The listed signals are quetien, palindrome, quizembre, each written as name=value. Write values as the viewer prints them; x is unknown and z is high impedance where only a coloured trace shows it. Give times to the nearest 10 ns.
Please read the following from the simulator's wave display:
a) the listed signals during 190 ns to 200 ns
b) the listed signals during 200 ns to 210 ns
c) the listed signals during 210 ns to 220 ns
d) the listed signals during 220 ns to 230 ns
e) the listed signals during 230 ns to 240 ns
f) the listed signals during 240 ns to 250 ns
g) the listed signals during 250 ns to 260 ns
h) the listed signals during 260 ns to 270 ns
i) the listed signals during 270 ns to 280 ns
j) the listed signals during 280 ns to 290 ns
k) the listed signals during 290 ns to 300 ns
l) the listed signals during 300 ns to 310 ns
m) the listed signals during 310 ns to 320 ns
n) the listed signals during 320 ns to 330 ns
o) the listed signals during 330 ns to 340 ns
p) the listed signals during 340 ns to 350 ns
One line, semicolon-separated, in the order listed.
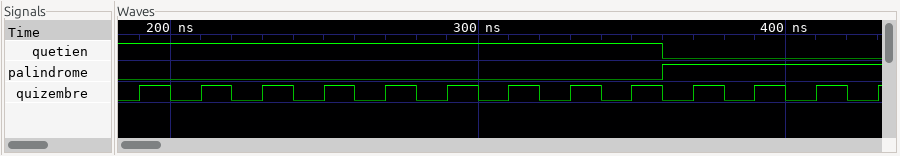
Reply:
quetien=1, palindrome=0, quizembre=1; quetien=1, palindrome=0, quizembre=0; quetien=1, palindrome=0, quizembre=1; quetien=1, palindrome=0, quizembre=0; quetien=1, palindrome=0, quizembre=1; quetien=1, palindrome=0, quizembre=0; quetien=1, palindrome=0, quizembre=1; quetien=1, palindrome=0, quizembre=0; quetien=1, palindrome=0, quizembre=1; quetien=1, palindrome=0, quizembre=0; quetien=1, palindrome=0, quizembre=1; quetien=1, palindrome=0, quizembre=0; quetien=1, palindrome=0, quizembre=1; quetien=1, palindrome=0, quizembre=0; quetien=1, palindrome=0, quizembre=1; quetien=1, palindrome=0, quizembre=0
